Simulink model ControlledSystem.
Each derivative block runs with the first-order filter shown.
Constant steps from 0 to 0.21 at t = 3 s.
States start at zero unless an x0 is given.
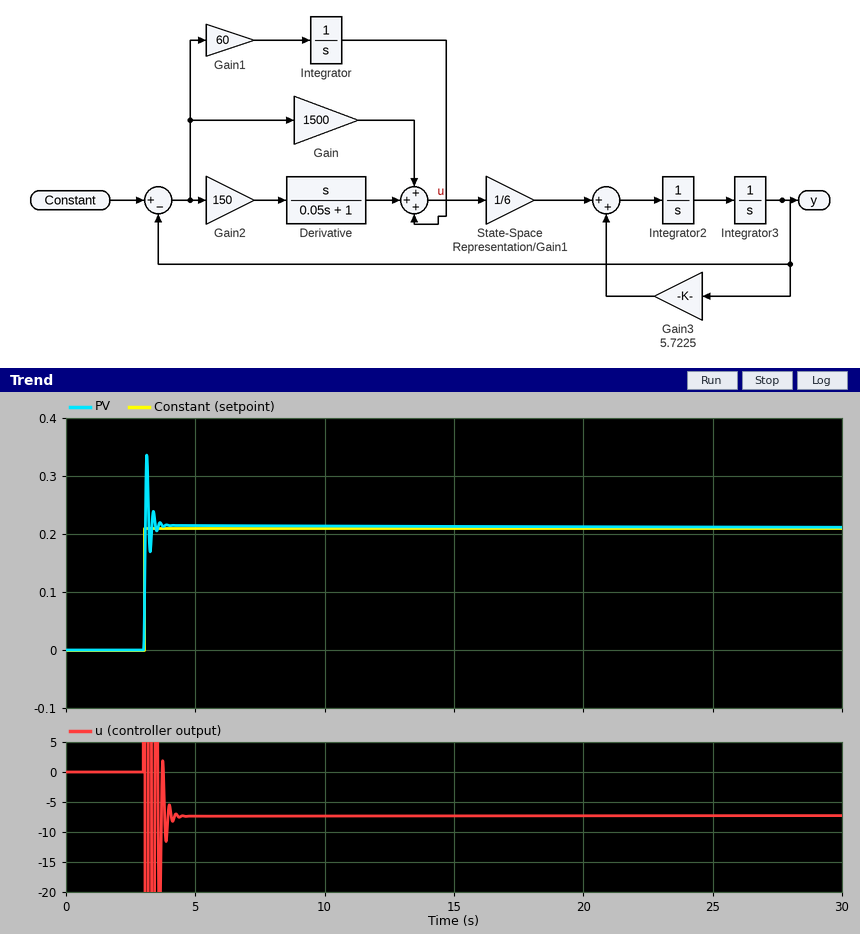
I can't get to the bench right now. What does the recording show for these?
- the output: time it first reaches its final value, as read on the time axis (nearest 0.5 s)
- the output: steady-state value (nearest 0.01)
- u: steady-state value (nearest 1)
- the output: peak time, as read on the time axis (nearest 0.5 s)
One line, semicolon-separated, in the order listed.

3.0 s; 0.21; -7; 3.0 s
